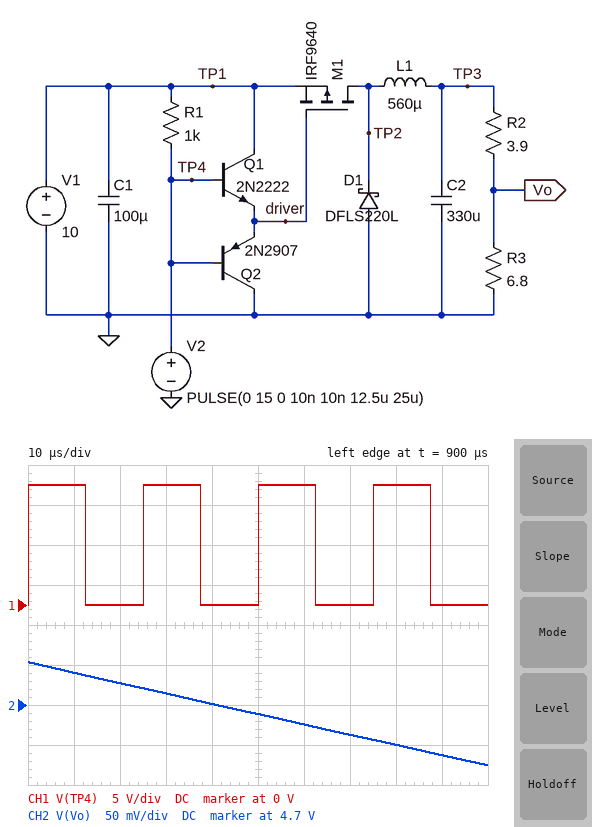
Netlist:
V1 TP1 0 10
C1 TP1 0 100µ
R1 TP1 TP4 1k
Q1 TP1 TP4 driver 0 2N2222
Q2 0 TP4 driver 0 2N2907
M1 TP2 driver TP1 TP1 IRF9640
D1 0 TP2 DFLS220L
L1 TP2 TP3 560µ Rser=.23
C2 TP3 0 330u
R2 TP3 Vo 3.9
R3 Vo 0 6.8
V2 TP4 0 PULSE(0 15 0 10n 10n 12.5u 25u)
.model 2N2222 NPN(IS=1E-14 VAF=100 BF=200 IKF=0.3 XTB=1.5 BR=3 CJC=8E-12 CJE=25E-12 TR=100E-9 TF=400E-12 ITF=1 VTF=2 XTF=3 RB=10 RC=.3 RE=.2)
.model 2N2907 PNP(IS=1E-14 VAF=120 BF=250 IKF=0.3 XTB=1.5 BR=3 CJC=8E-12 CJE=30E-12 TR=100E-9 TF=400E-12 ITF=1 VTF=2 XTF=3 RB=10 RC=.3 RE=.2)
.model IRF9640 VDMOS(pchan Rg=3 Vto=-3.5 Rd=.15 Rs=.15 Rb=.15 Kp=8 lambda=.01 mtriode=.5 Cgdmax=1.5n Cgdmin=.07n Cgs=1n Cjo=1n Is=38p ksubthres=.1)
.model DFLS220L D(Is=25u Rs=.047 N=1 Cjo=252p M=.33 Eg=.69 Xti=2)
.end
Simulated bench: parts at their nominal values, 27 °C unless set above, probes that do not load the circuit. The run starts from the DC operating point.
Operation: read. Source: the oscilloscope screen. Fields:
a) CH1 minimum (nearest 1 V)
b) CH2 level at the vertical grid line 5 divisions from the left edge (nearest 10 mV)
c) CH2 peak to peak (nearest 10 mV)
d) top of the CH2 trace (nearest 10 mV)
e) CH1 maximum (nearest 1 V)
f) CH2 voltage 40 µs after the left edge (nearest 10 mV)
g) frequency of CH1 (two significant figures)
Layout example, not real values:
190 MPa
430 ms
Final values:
0 V
4.69 V
130 mV
4.75 V
15 V
4.70 V
40 kHz
